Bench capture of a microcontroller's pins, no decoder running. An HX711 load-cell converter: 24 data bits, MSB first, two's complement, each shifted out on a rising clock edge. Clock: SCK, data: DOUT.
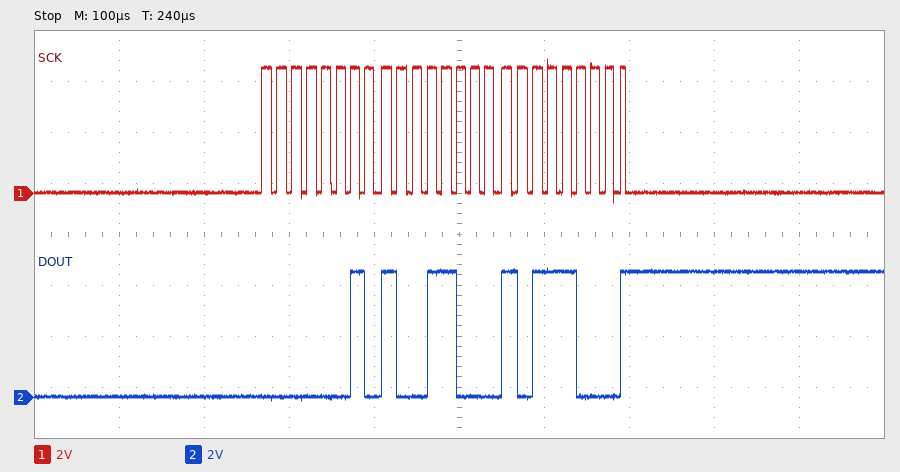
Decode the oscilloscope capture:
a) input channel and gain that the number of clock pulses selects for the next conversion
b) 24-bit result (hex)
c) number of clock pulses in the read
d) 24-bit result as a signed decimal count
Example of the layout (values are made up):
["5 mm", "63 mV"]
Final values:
["channel A, gain 128", "0x0298B8", "25", "170168"]
